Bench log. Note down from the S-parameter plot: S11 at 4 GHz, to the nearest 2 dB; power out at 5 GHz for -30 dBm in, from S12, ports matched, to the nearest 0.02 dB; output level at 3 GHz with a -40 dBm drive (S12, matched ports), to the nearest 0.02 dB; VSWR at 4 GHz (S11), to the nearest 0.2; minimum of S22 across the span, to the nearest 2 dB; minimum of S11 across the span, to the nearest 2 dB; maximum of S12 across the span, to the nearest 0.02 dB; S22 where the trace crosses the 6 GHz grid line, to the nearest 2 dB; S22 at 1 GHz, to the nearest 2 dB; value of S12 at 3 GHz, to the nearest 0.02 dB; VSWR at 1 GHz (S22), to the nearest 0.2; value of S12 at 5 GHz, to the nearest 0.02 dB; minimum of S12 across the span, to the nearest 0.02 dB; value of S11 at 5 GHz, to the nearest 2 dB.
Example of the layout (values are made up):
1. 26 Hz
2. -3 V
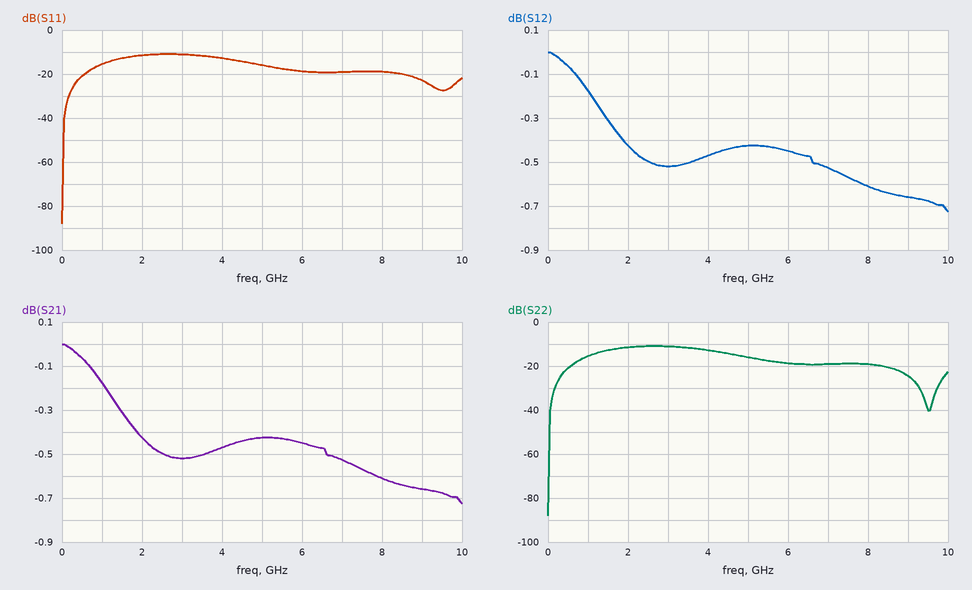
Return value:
1. -12 dB
2. -30.42 dBm
3. -40.52 dBm
4. 1.6
5. -88 dB
6. -88 dB
7. 0.00 dB
8. -18 dB
9. -16 dB
10. -0.52 dB
11. 1.4
12. -0.42 dB
13. -0.72 dB
14. -16 dB
